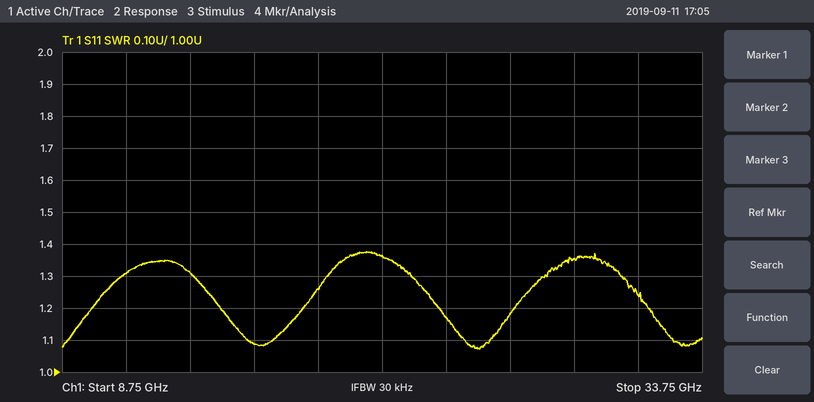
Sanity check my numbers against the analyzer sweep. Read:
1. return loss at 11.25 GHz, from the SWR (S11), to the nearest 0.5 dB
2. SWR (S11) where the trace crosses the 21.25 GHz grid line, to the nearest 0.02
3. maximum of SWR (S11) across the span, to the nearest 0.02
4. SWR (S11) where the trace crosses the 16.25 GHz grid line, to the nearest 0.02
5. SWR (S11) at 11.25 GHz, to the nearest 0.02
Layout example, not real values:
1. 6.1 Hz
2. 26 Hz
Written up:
1. 17.5 dB
2. 1.36
3. 1.38
4. 1.08
5. 1.30
